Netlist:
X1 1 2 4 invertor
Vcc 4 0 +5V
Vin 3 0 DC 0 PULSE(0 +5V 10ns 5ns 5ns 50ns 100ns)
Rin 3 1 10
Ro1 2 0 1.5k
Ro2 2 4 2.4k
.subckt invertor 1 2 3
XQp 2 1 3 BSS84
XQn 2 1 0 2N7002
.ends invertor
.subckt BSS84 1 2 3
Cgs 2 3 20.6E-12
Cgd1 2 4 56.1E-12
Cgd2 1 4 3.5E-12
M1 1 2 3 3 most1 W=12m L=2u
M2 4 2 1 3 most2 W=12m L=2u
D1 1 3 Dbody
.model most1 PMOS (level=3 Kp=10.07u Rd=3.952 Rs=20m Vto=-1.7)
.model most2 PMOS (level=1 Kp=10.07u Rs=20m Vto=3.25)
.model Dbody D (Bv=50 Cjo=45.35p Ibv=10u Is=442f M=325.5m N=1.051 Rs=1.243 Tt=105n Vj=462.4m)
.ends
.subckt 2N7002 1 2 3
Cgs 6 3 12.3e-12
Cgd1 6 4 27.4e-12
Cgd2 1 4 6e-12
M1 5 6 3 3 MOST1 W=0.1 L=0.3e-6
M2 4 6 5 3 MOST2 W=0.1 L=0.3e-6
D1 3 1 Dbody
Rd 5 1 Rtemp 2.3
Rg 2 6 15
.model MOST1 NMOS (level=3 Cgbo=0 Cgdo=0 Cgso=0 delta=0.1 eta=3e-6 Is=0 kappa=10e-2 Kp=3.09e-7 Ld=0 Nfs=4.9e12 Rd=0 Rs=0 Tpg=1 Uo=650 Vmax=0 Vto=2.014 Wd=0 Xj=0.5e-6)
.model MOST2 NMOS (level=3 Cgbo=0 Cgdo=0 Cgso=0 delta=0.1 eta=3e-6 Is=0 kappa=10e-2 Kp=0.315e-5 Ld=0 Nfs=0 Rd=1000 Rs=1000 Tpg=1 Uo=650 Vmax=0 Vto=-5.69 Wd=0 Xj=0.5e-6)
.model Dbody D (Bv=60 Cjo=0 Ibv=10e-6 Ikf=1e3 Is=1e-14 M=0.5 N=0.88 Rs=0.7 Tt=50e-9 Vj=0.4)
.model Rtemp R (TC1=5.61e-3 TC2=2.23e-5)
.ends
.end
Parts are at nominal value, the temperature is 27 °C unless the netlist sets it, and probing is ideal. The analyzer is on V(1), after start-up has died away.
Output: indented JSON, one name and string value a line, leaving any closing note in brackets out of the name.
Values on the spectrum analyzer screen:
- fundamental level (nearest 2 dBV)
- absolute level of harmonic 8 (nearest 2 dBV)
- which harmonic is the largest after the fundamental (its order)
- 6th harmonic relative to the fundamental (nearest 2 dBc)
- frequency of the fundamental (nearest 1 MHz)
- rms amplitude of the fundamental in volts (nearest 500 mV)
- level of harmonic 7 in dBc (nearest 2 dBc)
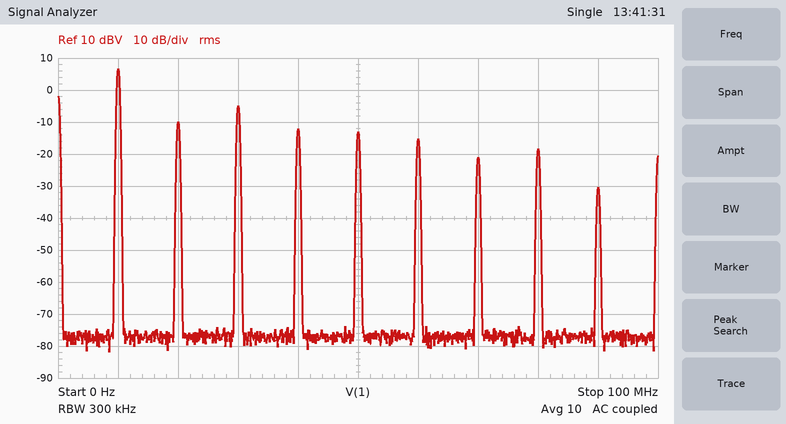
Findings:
{
  "fundamental level": "6 dBV",
  "absolute level of harmonic 8": "-18 dBV",
  "which harmonic is the largest after the fundamental": "3",
  "6th harmonic relative to the fundamental": "-22 dBc",
  "frequency of the fundamental": "10 MHz",
  "rms amplitude of the fundamental in volts": "2.0 V",
  "level of harmonic 7 in dBc": "-28 dBc"
}
